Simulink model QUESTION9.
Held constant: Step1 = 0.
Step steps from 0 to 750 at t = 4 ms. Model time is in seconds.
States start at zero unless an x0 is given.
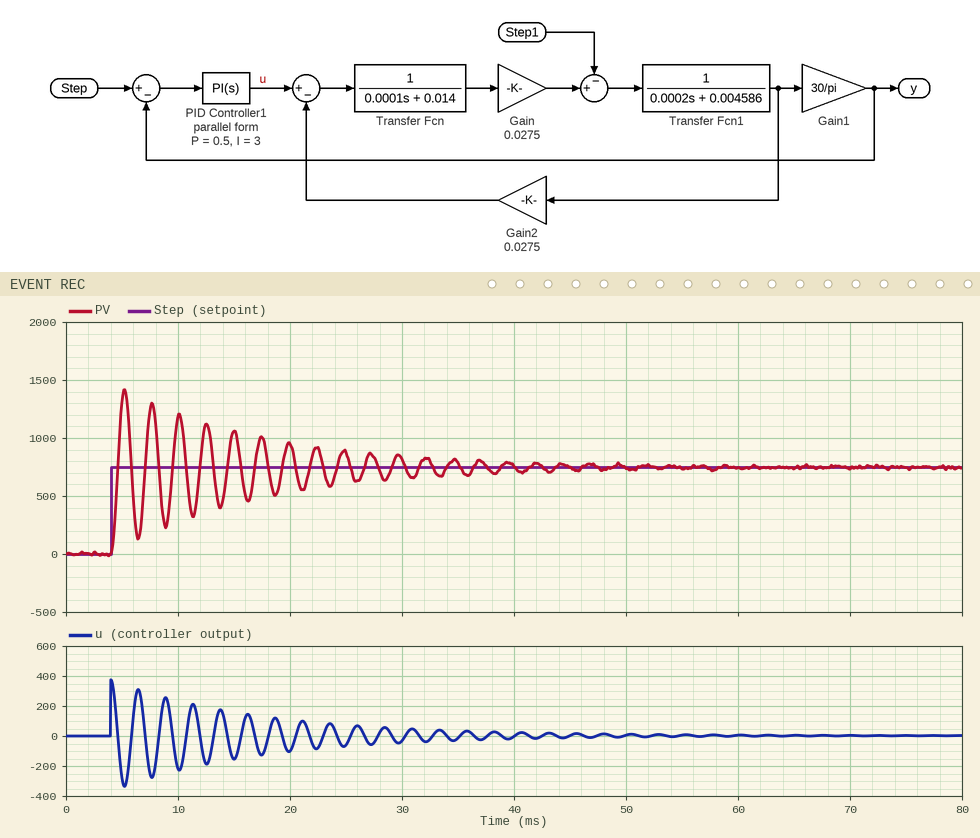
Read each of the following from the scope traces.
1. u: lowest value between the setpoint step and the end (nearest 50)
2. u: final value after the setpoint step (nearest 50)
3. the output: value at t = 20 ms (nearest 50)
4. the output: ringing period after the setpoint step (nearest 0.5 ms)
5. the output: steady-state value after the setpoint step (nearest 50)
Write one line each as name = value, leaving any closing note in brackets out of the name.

u: lowest value between the setpoint step and the end = -350
u: final value after the setpoint step = 0
the output: value at t = 20 ms = 950
the output: ringing period after the setpoint step = 2.5 ms
the output: steady-state value after the setpoint step = 750
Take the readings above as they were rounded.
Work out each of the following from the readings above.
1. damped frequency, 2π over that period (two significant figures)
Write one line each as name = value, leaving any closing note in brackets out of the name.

damped frequency, 2π over that period = 2.5 rad/ms
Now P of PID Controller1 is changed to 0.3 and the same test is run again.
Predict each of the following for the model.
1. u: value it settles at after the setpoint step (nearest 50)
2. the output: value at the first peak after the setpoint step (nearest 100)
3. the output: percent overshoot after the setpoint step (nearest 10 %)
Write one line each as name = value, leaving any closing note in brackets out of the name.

u: value it settles at after the setpoint step = 0
the output: value at the first peak after the setpoint step = 1400
the output: percent overshoot after the setpoint step = 90 %
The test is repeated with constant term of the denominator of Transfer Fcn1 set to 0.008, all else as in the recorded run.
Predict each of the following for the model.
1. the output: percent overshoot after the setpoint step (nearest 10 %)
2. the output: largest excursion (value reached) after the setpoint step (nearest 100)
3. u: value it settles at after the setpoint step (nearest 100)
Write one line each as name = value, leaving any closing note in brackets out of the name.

the output: percent overshoot after the setpoint step = 90 %
the output: largest excursion (value reached) after the setpoint step = 1400
u: value it settles at after the setpoint step = 0
